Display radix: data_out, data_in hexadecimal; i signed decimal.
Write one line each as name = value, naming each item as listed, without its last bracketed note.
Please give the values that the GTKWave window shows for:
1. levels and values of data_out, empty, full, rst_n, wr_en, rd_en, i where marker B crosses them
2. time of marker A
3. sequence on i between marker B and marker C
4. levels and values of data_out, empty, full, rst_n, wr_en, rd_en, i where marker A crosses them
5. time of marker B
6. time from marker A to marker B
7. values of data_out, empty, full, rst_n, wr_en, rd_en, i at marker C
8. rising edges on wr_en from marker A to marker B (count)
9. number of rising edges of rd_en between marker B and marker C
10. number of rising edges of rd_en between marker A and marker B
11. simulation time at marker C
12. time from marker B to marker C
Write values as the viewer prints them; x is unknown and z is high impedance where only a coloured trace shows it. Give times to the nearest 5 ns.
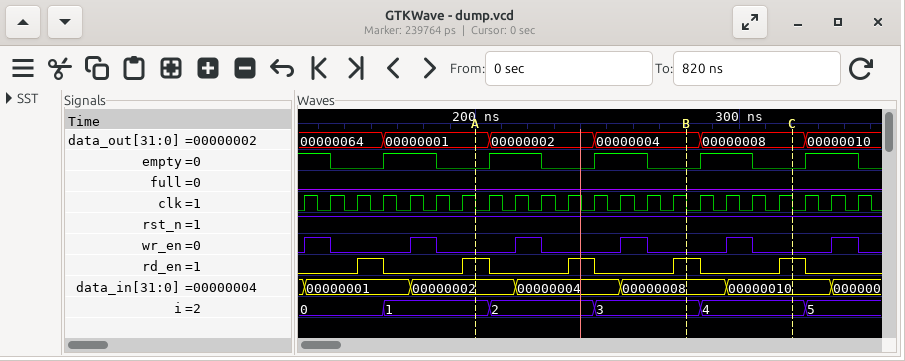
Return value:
levels and values of data_out, empty, full, rst_n, wr_en, rd_en, i where marker B crosses them = data_out=00000004, empty=0, full=0, rst_n=1, wr_en=0, rd_en=1, i=3
time of marker A = 200 ns
sequence on i between marker B and marker C = 3, 4
levels and values of data_out, empty, full, rst_n, wr_en, rd_en, i where marker A crosses them = data_out=00000001, empty=0, full=0, rst_n=1, wr_en=0, rd_en=1, i=1
time of marker B = 280 ns
time from marker A to marker B = 80 ns
values of data_out, empty, full, rst_n, wr_en, rd_en, i at marker C = data_out=00000008, empty=0, full=0, rst_n=1, wr_en=0, rd_en=1, i=4
rising edges on wr_en from marker A to marker B = 2
number of rising edges of rd_en between marker B and marker C = 1
number of rising edges of rd_en between marker A and marker B = 2
simulation time at marker C = 320 ns
time from marker B to marker C = 40 ns
